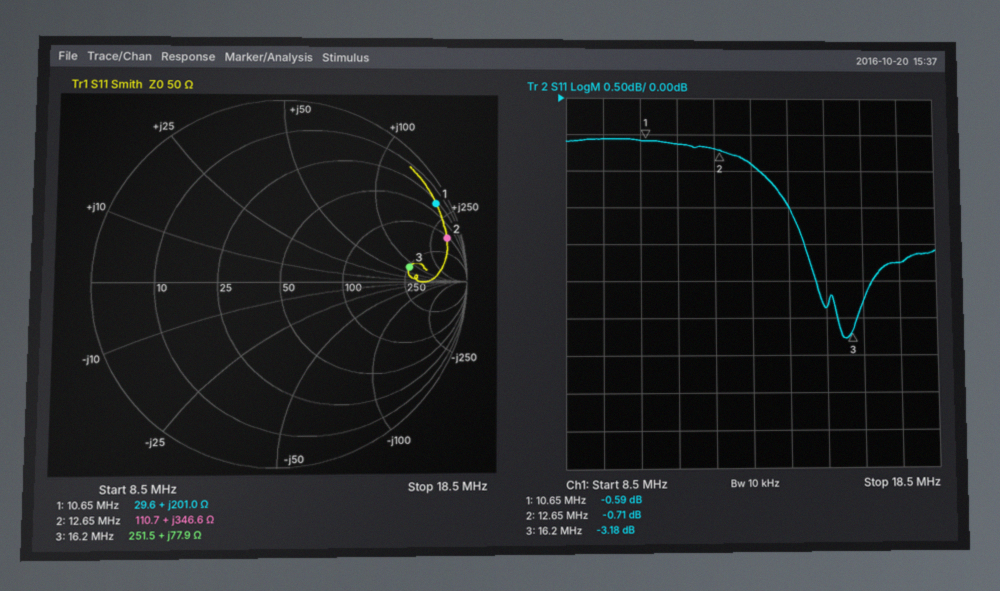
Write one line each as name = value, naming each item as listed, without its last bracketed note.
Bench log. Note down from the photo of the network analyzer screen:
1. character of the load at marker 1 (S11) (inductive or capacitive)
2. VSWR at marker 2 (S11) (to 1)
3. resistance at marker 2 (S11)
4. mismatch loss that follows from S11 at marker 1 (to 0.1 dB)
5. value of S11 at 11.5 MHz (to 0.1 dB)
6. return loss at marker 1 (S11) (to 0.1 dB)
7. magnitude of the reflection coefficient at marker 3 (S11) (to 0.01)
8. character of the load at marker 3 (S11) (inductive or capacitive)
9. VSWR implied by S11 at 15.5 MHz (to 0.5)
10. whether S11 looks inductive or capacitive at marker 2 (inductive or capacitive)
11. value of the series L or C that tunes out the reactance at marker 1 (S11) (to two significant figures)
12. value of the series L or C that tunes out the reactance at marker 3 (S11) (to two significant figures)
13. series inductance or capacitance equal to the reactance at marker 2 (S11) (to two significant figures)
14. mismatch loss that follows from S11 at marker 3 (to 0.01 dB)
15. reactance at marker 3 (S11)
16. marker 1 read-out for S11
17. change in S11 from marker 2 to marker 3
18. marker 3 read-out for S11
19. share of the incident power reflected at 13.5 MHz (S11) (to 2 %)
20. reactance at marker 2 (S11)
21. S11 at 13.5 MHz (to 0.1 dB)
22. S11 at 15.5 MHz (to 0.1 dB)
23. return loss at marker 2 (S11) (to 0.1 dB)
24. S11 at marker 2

character of the load at marker 1 (S11) = inductive
VSWR at marker 2 (S11) = 24
resistance at marker 2 = 110.7 Ω
mismatch loss that follows from S11 at marker 1 = 9.0 dB
value of S11 at 11.5 MHz = -0.6 dB
return loss at marker 1 (S11) = 0.6 dB
magnitude of the reflection coefficient at marker 3 (S11) = 0.69
character of the load at marker 3 (S11) = inductive
VSWR implied by S11 at 15.5 MHz = 6.0
whether S11 looks inductive or capacitive at marker 2 = inductive
value of the series L or C that tunes out the reactance at marker 1 (S11) = 74 pF
value of the series L or C that tunes out the reactance at marker 3 (S11) = 130 pF
series inductance or capacitance equal to the reactance at marker 2 (S11) = 4.4 µH
mismatch loss that follows from S11 at marker 3 = 2.85 dB
reactance at marker 3 = +77.9 Ω
marker 1 read-out for S11 = -0.59 dB
change in S11 from marker 2 to marker 3 = -2.47 dB
marker 3 read-out for S11 = -3.18 dB
share of the incident power reflected at 13.5 MHz (S11) = 82 %
reactance at marker 2 = +346.6 Ω
S11 at 13.5 MHz = -0.9 dB
S11 at 15.5 MHz = -2.9 dB
return loss at marker 2 (S11) = 0.7 dB
S11 at marker 2 = -0.71 dB
